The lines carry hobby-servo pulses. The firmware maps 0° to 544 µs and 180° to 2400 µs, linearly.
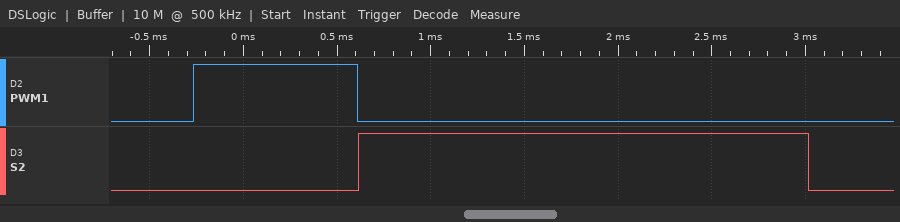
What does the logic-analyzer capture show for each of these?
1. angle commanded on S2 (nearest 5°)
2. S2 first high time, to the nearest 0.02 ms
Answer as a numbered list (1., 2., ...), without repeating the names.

1. 180°
2. 2.40 ms
